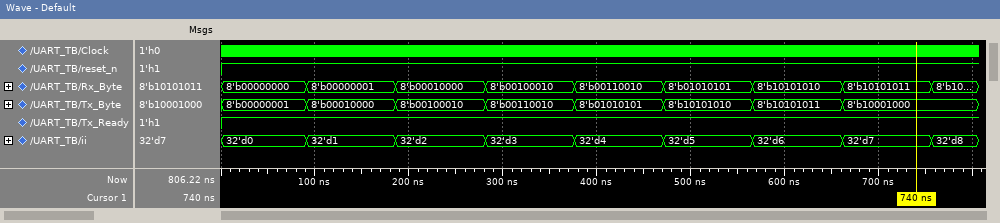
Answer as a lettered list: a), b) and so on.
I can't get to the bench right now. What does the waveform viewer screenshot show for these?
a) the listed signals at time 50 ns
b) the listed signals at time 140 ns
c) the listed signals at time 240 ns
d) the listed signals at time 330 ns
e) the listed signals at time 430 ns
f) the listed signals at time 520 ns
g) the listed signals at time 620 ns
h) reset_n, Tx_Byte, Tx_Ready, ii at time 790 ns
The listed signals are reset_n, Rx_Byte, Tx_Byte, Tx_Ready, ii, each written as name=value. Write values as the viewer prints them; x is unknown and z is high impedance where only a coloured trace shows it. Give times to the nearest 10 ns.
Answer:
a) reset_n=1, Rx_Byte=8'b00000000, Tx_Byte=8'b00000001, Tx_Ready=1, ii=32'd0
b) reset_n=1, Rx_Byte=8'b00000001, Tx_Byte=8'b00010000, Tx_Ready=1, ii=32'd1
c) reset_n=1, Rx_Byte=8'b00010000, Tx_Byte=8'b00100010, Tx_Ready=1, ii=32'd2
d) reset_n=1, Rx_Byte=8'b00100010, Tx_Byte=8'b00110010, Tx_Ready=1, ii=32'd3
e) reset_n=1, Rx_Byte=8'b00110010, Tx_Byte=8'b01010101, Tx_Ready=1, ii=32'd4
f) reset_n=1, Rx_Byte=8'b01010101, Tx_Byte=8'b10101010, Tx_Ready=1, ii=32'd5
g) reset_n=1, Rx_Byte=8'b10101010, Tx_Byte=8'b10101011, Tx_Ready=1, ii=32'd6
h) reset_n=1, Tx_Byte=8'b10001000, Tx_Ready=1, ii=32'd8
